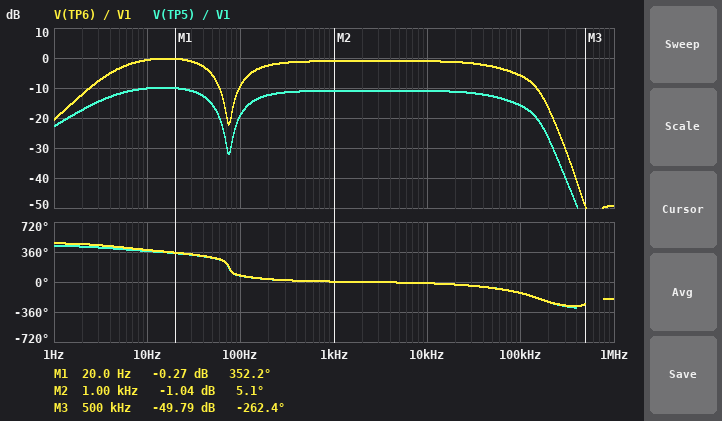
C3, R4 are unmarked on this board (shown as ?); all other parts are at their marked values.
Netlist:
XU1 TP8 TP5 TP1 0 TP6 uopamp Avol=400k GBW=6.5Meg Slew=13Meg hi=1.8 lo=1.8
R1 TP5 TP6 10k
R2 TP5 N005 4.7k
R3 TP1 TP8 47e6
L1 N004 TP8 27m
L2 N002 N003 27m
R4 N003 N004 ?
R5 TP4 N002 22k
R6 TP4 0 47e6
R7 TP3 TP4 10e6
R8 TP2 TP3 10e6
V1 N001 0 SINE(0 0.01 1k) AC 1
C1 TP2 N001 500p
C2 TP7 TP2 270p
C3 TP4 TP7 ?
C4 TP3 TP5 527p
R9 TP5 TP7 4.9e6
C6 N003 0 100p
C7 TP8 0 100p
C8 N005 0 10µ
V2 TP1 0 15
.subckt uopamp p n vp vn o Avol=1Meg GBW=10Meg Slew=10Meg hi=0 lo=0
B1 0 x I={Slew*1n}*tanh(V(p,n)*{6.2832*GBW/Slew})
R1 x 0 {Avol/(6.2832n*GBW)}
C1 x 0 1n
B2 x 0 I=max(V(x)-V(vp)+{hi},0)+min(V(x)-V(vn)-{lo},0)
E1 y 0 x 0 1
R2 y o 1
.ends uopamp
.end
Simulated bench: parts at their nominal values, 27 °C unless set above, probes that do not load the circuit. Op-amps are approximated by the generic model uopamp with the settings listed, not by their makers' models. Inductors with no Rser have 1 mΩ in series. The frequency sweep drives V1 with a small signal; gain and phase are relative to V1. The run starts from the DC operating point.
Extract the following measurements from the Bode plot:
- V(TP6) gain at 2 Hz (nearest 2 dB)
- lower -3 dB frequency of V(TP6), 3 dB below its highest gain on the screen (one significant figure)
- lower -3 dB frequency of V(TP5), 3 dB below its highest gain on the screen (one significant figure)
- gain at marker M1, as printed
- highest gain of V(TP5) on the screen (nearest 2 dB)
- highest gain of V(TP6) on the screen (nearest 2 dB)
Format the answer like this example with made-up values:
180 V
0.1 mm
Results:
-12 dB
5 Hz
4 Hz
-0.27 dB
-10 dB
0 dB
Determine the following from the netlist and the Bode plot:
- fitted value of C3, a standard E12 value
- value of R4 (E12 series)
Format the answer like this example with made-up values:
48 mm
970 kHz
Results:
150 pF
47 kΩ
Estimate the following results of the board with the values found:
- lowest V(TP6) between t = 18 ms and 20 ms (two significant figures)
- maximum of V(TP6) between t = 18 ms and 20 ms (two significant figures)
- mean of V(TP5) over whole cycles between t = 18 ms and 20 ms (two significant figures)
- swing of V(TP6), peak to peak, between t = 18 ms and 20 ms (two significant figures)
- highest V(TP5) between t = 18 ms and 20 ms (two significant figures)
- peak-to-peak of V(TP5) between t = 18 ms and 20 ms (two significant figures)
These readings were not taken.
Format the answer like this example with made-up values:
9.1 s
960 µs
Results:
7.5 V
7.5 V
7.5 V
18 mV
7.5 V
5.7 mV
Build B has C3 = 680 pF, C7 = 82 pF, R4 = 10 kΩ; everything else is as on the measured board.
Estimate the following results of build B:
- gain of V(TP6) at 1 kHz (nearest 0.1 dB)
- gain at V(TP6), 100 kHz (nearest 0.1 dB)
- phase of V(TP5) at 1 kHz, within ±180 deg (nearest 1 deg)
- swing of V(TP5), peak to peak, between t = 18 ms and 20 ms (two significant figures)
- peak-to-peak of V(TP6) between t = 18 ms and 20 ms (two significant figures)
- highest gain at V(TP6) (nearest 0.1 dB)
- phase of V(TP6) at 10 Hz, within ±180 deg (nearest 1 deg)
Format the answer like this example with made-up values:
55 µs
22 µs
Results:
2.6 dB
4.4 dB
2 deg
8.6 mV
27 mV
4.7 dB
26 deg
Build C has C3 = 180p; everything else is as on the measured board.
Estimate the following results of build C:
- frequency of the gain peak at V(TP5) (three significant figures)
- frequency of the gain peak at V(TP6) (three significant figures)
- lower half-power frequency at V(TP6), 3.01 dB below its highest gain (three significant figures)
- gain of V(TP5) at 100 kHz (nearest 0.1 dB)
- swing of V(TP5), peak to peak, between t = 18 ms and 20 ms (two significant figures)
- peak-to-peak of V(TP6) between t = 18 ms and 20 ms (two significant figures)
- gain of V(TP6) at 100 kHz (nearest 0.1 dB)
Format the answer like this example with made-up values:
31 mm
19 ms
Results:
14.4 Hz
15.9 Hz
5.19 Hz
-15.6 dB
6.1 mV
19 mV
-5.7 dB
